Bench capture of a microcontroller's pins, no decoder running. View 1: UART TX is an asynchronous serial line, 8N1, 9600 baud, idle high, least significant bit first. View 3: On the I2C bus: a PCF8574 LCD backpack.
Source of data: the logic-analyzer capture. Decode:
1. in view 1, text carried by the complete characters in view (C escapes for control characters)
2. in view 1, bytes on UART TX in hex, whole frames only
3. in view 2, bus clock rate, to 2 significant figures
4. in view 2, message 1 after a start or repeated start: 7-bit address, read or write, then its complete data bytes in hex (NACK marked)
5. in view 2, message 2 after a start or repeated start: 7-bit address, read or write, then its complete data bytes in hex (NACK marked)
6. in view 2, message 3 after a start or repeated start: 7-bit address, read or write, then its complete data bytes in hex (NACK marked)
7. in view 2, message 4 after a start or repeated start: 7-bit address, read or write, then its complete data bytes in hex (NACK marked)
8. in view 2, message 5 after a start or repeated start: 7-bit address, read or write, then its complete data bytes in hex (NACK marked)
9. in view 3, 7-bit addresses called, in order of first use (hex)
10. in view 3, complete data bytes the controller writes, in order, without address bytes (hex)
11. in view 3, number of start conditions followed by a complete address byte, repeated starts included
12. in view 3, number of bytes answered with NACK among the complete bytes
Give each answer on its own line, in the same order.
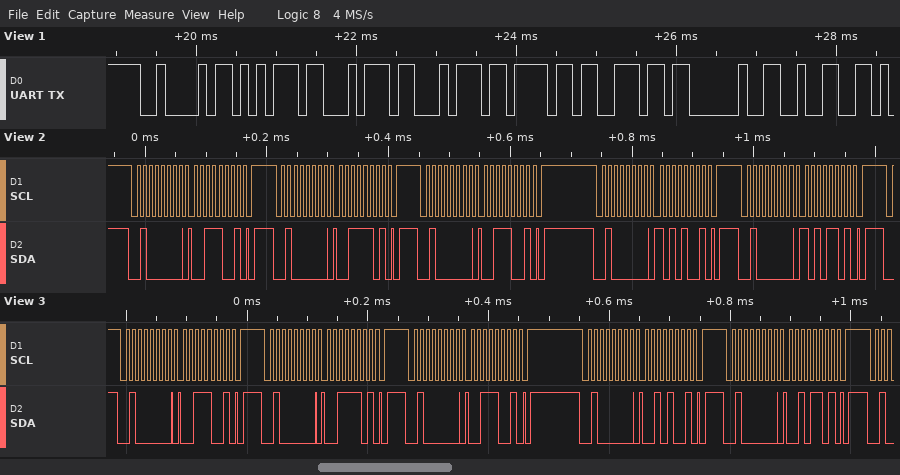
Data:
"Button 2"
42 75 74 74 6F 6E 20 32
100 kHz
0x20 write: 39
0x20 write: 3D
0x20 write: 39
0x20 write: A9
0x20 write: AD
0x20
39 3D 39 29 2D
5
0
